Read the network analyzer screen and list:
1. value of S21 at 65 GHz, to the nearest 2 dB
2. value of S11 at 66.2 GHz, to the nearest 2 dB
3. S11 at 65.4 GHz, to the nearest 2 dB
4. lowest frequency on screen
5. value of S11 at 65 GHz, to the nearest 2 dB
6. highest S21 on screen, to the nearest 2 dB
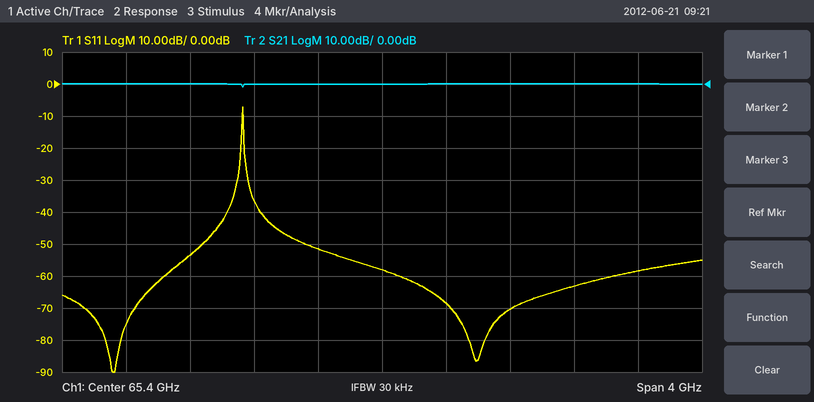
0 dB
-70 dB
-58 dB
63.4 GHz
-52 dB
0 dB
